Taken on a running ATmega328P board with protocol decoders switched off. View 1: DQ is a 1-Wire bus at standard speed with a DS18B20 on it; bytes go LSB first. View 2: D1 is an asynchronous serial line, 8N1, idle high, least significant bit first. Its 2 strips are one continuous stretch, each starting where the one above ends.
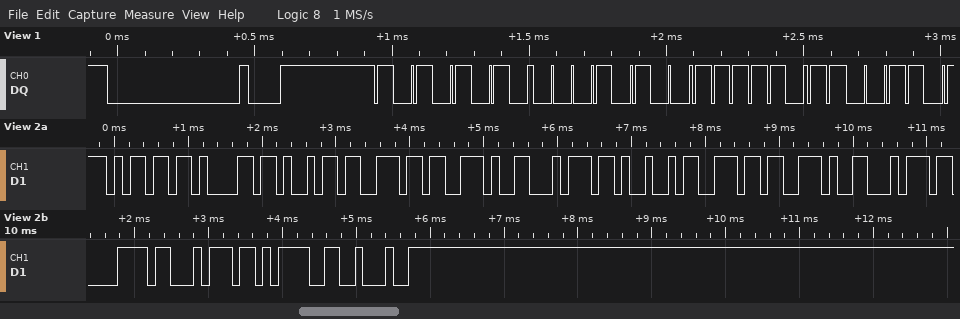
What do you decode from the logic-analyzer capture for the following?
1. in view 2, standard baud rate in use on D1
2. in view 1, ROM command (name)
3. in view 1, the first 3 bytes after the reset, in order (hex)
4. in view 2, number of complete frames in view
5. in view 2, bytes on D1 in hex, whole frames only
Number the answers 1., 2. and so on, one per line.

1. 9600 baud
2. Match ROM
3. 55 28 DF
4. 14
5. 6D 61 69 6E 2E 74 49 6E 2E 74 78 74 3D 22
